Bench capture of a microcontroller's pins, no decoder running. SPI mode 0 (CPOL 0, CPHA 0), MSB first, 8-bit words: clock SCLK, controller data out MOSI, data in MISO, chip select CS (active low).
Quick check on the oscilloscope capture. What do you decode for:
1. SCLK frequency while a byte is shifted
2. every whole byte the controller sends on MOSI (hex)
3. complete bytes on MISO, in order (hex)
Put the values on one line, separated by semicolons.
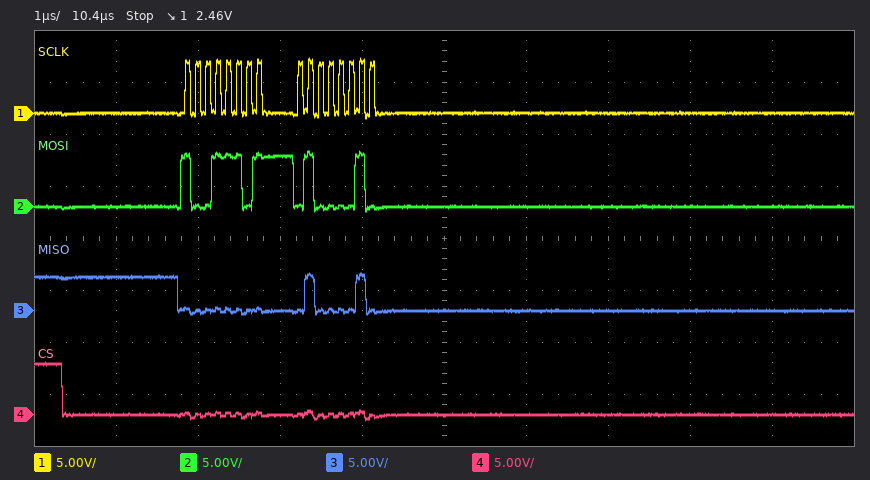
8 MHz; 9D 42; 00 42
